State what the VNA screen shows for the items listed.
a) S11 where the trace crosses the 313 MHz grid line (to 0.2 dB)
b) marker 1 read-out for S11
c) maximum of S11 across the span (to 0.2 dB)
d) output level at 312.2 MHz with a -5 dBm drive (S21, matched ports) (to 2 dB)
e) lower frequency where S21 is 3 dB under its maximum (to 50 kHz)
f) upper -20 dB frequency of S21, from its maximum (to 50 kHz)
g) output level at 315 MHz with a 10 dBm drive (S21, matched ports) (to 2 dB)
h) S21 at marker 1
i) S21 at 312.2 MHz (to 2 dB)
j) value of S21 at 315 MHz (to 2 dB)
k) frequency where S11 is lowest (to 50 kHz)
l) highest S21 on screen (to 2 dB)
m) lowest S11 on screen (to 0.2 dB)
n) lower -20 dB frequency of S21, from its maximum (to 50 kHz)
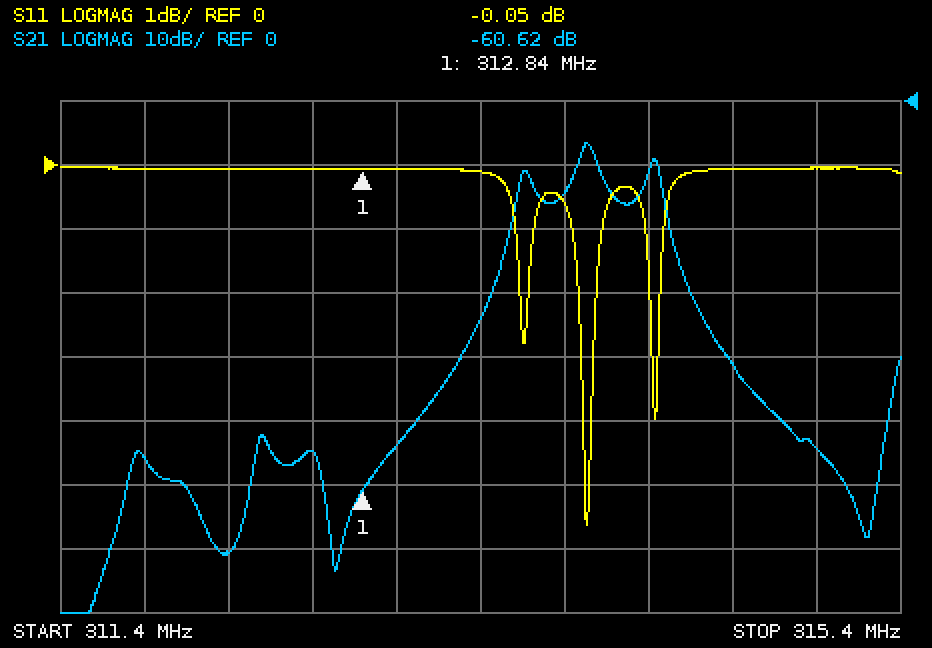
0.0 dB
-0.05 dB
0.0 dB
-76 dBm
313.85 MHz
314.35 MHz
-44 dBm
-60.62 dB
-70 dB
-54 dB
313.90 MHz
-6 dB
-5.6 dB
313.50 MHz
